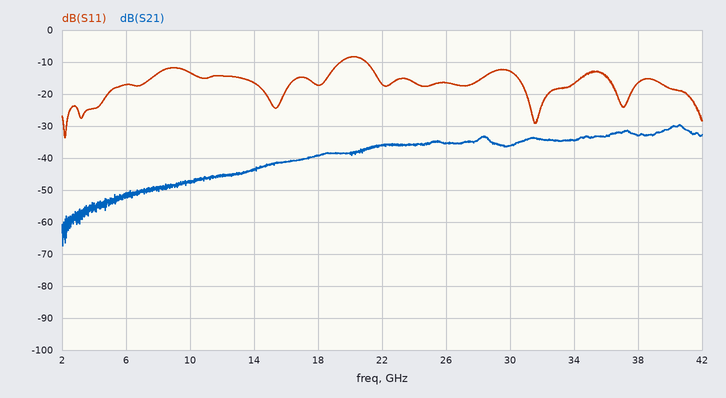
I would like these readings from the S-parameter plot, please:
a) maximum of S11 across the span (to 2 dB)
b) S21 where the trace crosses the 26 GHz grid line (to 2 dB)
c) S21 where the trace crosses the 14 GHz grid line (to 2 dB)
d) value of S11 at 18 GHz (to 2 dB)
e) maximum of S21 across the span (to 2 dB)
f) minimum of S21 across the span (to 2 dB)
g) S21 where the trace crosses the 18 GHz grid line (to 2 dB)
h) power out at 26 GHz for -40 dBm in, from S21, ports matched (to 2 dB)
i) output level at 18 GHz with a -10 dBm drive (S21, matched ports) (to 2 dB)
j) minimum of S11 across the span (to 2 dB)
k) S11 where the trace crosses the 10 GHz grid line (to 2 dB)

-8 dB
-36 dB
-44 dB
-18 dB
-30 dB
-68 dB
-40 dB
-76 dBm
-50 dBm
-34 dB
-14 dB
